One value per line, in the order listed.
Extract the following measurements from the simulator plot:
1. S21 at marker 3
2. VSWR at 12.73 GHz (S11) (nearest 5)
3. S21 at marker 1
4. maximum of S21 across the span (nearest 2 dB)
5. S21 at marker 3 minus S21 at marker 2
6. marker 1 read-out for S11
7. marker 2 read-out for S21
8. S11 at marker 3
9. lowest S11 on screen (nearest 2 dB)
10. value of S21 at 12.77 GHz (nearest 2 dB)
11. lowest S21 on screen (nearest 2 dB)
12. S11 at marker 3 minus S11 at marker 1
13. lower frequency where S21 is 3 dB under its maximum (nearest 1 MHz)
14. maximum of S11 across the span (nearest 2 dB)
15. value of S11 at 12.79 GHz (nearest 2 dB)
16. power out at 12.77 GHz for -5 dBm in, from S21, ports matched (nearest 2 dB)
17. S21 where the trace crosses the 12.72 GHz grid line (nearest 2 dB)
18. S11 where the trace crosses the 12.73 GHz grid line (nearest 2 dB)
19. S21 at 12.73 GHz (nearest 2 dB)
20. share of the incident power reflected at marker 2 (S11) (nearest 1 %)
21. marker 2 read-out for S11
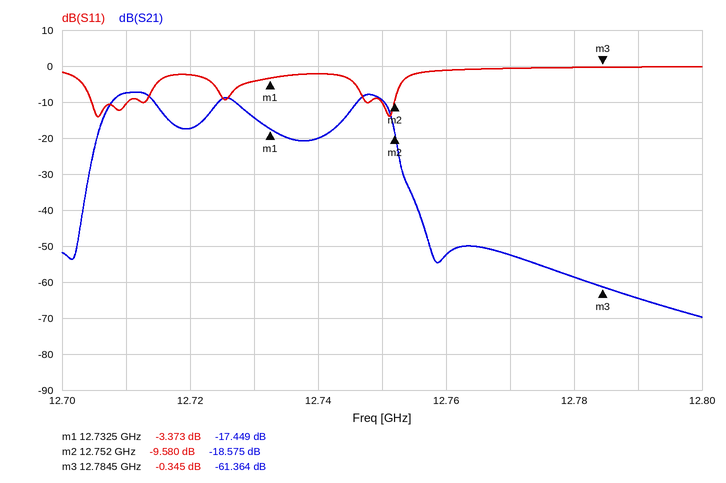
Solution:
-61.364 dB
5
-17.449 dB
-8 dB
-42.789 dB
-3.373 dB
-18.575 dB
-0.345 dB
-14 dB
-52 dB
-70 dB
3.028 dB
12.708 GHz
0 dB
0 dB
-58 dBm
-18 dB
-4 dB
-14 dB
11 %
-9.580 dB
